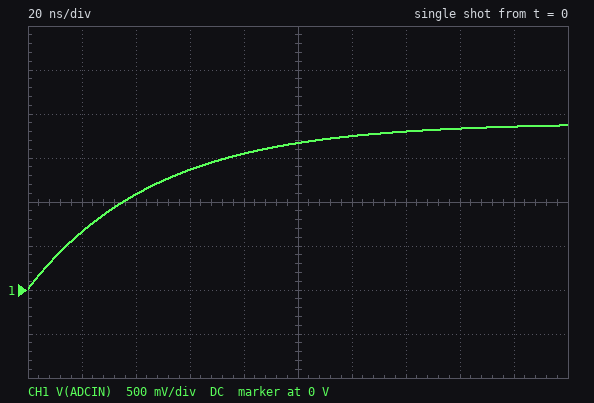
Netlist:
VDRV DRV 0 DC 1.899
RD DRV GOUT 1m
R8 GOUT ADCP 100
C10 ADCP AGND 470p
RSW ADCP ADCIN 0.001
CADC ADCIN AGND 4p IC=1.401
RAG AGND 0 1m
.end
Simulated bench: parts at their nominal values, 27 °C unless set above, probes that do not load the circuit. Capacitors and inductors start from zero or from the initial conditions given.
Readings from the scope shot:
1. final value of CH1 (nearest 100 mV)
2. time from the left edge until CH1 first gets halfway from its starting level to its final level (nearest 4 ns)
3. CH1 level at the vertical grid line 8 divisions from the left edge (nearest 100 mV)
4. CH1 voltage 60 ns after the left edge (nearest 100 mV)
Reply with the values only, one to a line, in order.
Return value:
1.9 V
32 ns
1.8 V
1.4 V
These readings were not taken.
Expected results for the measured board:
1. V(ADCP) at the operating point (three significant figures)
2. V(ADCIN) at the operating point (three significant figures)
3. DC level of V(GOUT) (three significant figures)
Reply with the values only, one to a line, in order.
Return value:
1.90 V
1.90 V
1.90 V
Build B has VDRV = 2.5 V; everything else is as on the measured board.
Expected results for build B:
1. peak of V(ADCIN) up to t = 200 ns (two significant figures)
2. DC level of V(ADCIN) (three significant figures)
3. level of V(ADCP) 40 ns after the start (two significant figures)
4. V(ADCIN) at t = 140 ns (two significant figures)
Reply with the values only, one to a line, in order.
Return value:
2.5 V
2.50 V
1.4 V
2.4 V
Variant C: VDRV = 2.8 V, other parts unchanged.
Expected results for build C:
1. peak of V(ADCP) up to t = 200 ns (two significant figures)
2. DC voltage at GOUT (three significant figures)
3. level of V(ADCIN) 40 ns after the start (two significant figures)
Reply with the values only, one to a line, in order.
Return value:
2.8 V
2.80 V
1.6 V
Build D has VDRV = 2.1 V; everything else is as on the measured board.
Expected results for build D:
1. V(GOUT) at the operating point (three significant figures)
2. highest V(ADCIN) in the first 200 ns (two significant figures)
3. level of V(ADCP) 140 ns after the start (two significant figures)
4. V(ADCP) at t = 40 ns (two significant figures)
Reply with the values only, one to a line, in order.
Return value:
2.10 V
2.1 V
2.0 V
1.2 V
